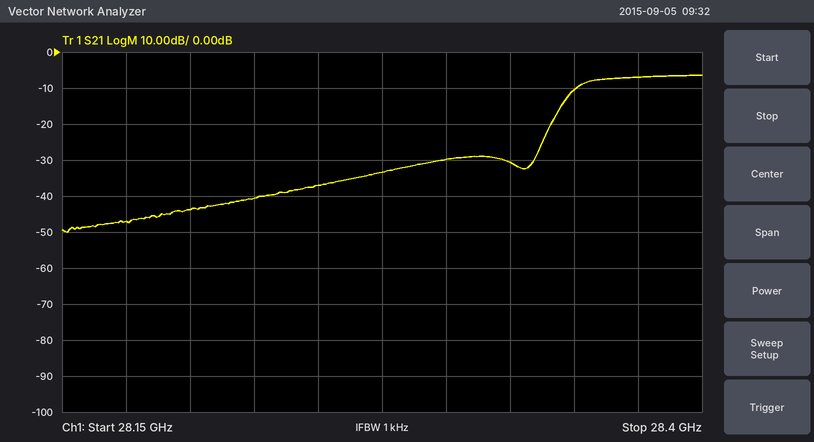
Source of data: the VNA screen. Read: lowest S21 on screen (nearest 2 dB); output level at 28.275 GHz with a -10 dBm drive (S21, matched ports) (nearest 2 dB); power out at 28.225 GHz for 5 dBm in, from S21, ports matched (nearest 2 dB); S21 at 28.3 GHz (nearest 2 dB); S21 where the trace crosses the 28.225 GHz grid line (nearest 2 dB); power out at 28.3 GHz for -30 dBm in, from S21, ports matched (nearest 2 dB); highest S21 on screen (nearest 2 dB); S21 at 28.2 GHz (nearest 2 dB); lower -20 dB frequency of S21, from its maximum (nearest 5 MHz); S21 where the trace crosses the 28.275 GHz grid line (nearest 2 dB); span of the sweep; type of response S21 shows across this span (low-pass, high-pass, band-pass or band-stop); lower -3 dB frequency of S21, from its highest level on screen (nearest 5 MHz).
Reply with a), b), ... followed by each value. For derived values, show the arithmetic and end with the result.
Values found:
a) -50 dB
b) -10 dBm + (-34 dB) = -44 dBm
c) 5 dBm + (-40 dB) = -36 dBm
d) -30 dB
e) -40 dB
f) -30 dBm + (-30 dB) = -60 dBm
g) -6 dB
h) -44 dB
i) 28.335 GHz
j) -34 dB
k) 250 MHz
l) high-pass
m) 28.350 GHz
